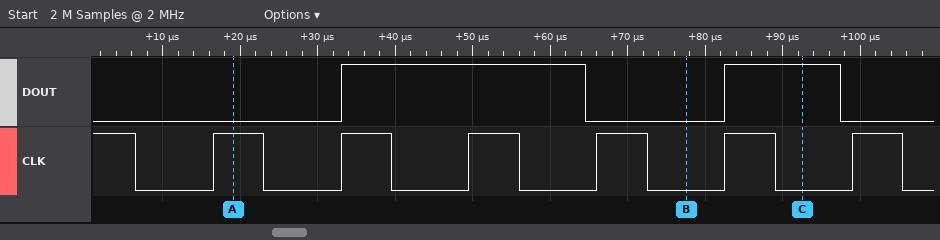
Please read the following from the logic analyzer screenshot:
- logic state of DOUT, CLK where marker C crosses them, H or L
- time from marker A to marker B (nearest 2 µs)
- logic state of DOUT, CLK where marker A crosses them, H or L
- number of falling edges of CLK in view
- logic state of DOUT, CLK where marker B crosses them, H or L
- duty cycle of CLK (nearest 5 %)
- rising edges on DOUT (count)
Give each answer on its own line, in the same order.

DOUT=H, CLK=L
58 µs
DOUT=L, CLK=H
7
DOUT=L, CLK=L
40 %
2
